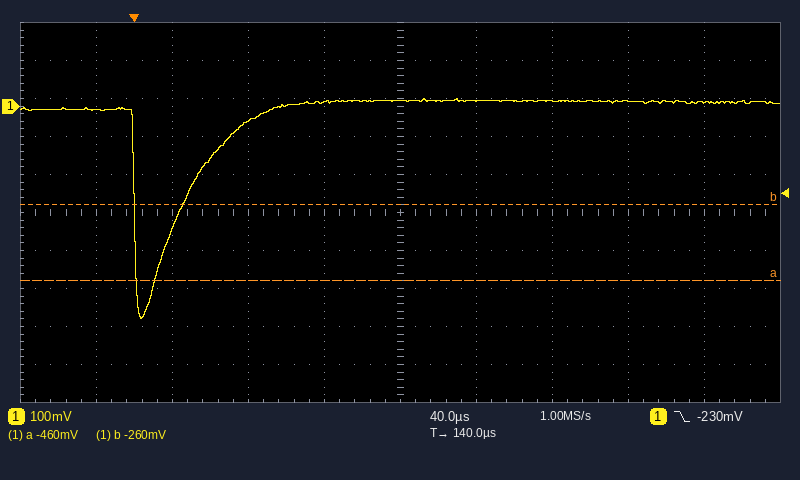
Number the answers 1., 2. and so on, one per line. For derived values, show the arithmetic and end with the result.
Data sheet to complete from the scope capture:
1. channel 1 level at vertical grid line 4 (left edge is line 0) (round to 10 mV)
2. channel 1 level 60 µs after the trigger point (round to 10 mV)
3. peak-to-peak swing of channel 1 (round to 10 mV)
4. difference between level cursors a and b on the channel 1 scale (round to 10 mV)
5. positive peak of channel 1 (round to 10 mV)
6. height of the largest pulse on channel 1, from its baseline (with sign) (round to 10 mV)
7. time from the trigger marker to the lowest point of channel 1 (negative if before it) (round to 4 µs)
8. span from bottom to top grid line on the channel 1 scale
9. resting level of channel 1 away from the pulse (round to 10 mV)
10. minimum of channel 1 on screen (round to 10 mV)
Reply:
1. 10 mV
2. -40 mV
3. 20 mV − (-560 mV) = 580 mV
4. 200 mV
5. 20 mV
6. -560 mV − (10 mV) = -570 mV
7. +4 µs
8. 1 V
9. 10 mV
10. -560 mV
